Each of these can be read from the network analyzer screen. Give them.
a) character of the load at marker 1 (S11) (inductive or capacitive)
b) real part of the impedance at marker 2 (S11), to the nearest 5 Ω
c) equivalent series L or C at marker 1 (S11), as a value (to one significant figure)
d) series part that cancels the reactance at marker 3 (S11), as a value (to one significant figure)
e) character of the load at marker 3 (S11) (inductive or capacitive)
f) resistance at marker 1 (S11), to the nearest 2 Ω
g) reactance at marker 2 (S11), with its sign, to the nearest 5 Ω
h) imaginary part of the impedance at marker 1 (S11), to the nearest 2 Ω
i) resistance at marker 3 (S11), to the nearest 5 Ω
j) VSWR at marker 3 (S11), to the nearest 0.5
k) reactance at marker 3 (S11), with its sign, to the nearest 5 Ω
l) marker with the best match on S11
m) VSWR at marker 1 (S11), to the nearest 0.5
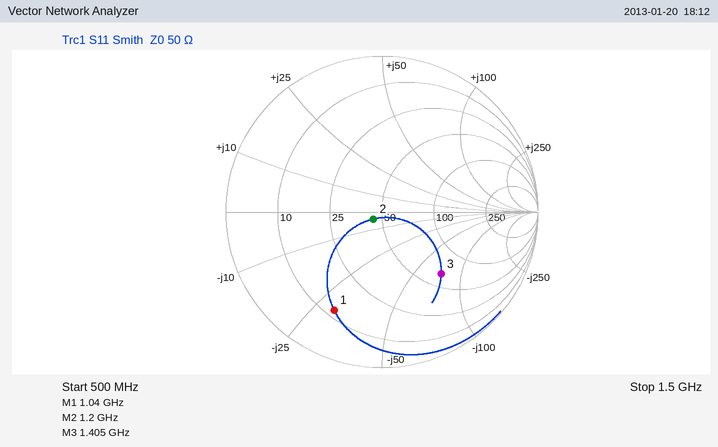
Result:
capacitive
45 Ω
5 pF
8 nH
capacitive
12 Ω
-5 Ω
-30 Ω
65 Ω
3.5
-75 Ω
marker 2
5.5
